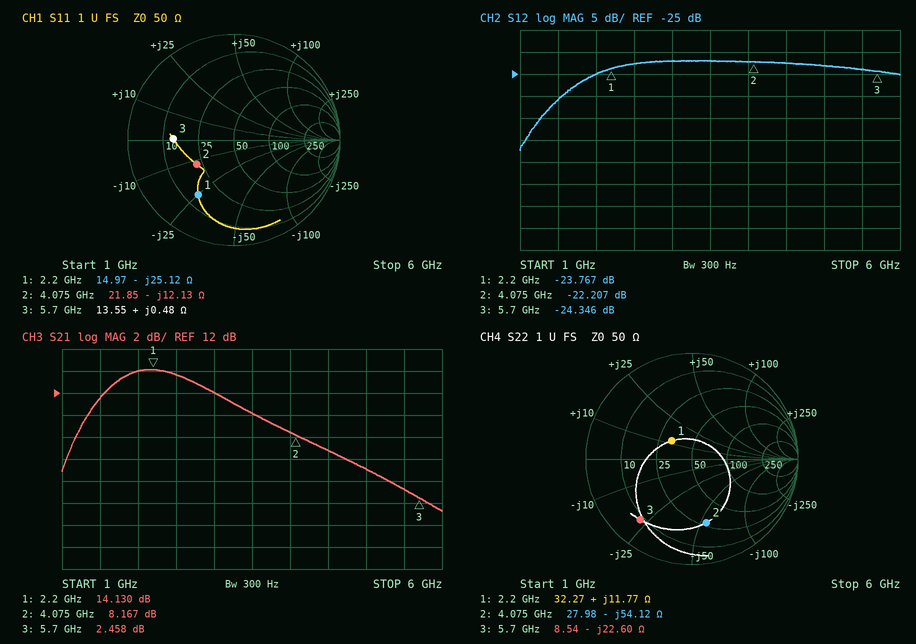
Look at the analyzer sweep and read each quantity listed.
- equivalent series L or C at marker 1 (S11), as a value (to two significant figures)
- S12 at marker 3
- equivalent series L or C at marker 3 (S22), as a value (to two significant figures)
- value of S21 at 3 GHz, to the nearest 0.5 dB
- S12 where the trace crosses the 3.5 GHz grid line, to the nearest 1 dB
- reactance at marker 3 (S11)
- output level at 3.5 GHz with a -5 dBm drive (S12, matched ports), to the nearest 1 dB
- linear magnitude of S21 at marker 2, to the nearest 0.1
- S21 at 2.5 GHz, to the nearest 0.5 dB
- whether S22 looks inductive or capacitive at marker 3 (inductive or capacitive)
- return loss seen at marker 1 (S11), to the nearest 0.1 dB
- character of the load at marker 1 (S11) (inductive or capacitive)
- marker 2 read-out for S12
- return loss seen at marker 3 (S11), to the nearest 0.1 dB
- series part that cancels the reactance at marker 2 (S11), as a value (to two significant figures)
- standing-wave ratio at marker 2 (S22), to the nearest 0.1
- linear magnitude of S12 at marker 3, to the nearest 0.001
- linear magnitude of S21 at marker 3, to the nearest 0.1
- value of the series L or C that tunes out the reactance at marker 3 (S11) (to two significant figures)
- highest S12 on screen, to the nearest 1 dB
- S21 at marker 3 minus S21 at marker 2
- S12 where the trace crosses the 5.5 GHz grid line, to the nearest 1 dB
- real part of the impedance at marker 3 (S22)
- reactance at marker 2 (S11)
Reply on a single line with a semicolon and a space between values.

2.9 pF; -24.346 dB; 1.2 pF; 12.0 dB; -22 dB; +0.48 Ω; -27 dBm; 2.6; 13.5 dB; capacitive; 4.2 dB; capacitive; -22.207 dB; 4.8 dB; 470 pH; 4.2; 0.061; 1.3; 58 pF; -22 dB; -5.709 dB; -24 dB; 8.54 Ω; -12.13 Ω
